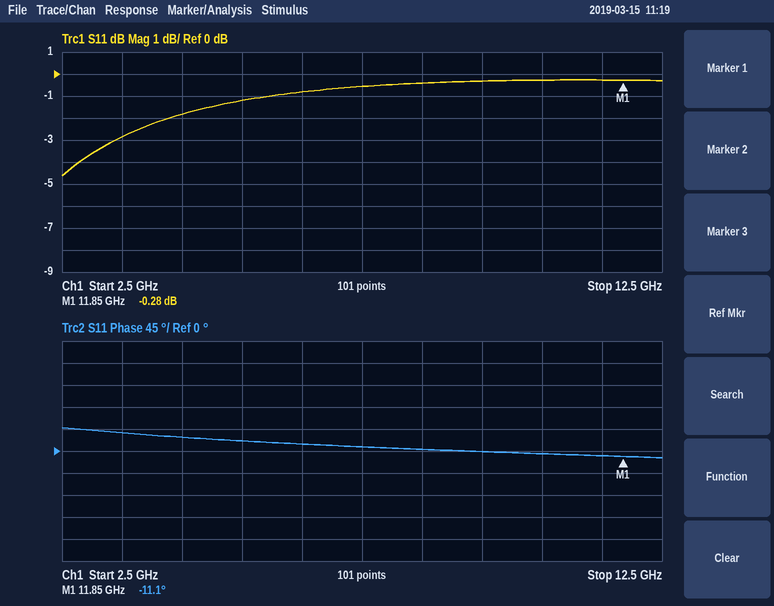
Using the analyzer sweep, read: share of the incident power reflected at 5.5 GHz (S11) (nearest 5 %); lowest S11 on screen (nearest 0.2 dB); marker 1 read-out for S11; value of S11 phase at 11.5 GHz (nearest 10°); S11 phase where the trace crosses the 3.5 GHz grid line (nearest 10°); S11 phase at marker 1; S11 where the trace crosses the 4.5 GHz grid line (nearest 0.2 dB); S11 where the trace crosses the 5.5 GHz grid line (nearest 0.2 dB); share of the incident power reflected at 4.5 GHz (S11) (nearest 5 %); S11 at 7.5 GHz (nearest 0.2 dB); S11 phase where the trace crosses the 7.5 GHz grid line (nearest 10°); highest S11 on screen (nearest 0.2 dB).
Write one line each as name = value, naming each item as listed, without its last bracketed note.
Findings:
share of the incident power reflected at 5.5 GHz (S11) = 75 %
lowest S11 on screen = -4.6 dB
marker 1 read-out for S11 = -0.28 dB
value of S11 phase at 11.5 GHz = -10°
S11 phase where the trace crosses the 3.5 GHz grid line = 40°
S11 phase at marker 1 = -11.1°
S11 where the trace crosses the 4.5 GHz grid line = -1.8 dB
S11 where the trace crosses the 5.5 GHz grid line = -1.2 dB
share of the incident power reflected at 4.5 GHz (S11) = 65 %
S11 at 7.5 GHz = -0.6 dB
S11 phase where the trace crosses the 7.5 GHz grid line = 10°
highest S11 on screen = -0.2 dB
